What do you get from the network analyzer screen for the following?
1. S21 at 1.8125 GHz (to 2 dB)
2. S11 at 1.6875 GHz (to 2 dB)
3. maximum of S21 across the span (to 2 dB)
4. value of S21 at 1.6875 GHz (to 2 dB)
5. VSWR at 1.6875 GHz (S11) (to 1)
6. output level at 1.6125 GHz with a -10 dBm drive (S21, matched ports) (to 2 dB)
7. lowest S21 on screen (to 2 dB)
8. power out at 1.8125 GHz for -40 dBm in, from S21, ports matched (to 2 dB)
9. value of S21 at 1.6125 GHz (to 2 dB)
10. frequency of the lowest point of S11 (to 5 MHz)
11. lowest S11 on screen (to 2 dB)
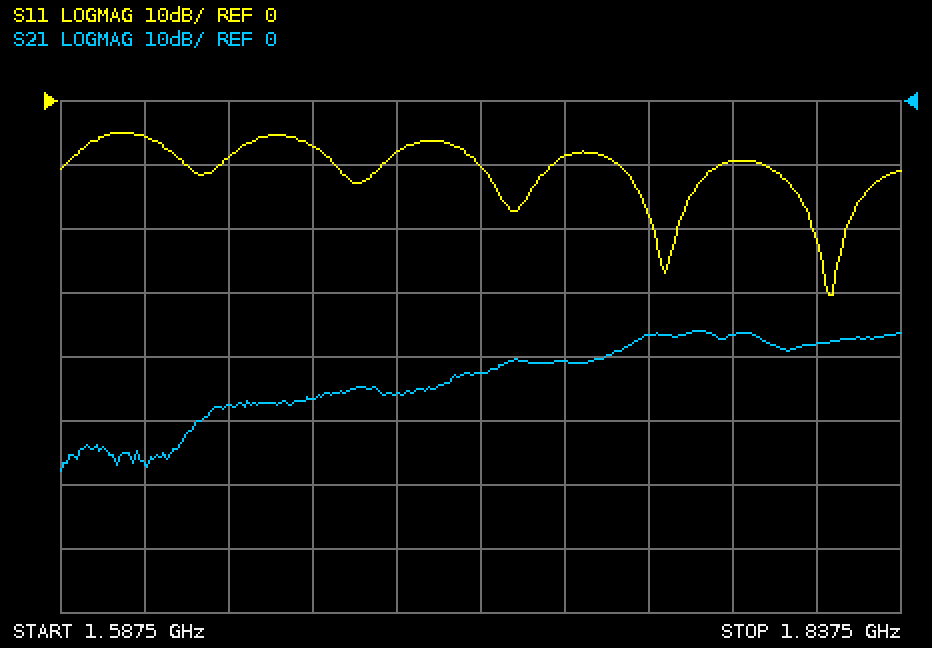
-38 dB
-8 dB
-36 dB
-46 dB
2
-66 dBm
-58 dB
-78 dBm
-56 dB
1.815 GHz
-30 dB
